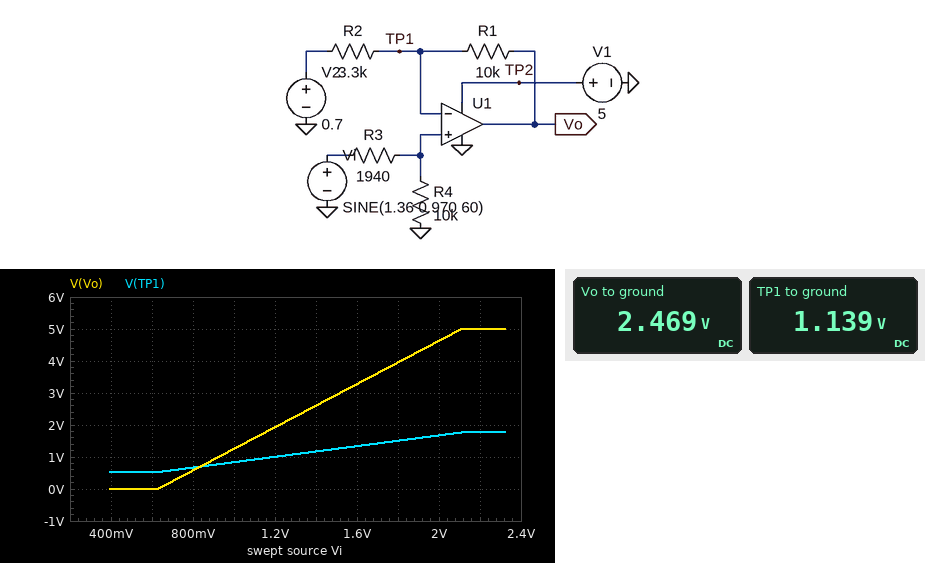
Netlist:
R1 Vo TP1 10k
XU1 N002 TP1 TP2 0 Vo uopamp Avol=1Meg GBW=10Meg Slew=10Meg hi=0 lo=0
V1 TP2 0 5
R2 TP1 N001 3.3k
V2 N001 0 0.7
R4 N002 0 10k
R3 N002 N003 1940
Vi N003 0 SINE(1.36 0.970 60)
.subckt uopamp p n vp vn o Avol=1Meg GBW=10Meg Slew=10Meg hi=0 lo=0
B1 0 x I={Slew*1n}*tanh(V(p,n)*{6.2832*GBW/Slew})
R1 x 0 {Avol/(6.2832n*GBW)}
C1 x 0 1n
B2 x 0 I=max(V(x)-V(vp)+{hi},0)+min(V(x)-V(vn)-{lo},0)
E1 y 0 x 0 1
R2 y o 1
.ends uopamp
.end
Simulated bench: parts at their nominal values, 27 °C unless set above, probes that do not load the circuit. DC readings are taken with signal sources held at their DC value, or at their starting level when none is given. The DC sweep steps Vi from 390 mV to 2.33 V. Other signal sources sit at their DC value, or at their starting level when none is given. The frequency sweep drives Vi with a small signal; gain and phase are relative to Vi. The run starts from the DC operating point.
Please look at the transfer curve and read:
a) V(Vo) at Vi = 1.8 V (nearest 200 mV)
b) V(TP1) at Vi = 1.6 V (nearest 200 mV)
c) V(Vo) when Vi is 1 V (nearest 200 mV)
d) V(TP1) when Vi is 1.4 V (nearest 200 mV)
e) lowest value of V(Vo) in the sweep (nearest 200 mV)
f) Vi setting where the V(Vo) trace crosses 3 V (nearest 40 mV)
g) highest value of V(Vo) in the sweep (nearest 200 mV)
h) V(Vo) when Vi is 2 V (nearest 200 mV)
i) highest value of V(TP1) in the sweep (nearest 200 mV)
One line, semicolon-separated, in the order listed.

4.0 V; 1.4 V; 1.2 V; 1.2 V; 0 V; 1.52 V; 5.0 V; 4.6 V; 1.8 V
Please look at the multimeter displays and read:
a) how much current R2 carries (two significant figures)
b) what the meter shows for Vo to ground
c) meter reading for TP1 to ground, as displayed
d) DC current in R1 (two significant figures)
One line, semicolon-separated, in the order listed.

130 µA; 2.469 V; 1.139 V; 130 µA
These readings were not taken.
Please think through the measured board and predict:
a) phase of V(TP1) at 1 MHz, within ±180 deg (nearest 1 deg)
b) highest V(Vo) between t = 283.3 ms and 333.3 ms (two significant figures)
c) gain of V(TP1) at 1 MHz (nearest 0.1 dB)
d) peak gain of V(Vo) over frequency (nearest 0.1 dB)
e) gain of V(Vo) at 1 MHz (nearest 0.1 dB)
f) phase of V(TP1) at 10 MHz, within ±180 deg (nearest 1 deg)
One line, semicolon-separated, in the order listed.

-22 deg; 5.0 V; -2.2 dB; 10.6 dB; 9.9 dB; -76 deg
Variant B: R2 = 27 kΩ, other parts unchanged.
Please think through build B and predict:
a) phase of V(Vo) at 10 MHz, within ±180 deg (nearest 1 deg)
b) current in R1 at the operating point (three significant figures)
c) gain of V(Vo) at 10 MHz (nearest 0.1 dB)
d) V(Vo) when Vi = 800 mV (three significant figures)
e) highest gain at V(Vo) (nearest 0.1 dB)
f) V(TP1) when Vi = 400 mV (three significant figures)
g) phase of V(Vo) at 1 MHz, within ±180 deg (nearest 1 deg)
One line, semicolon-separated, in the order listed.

-54 deg; 16.3 µA; -3.4 dB; 659 mV; 1.2 dB; 335 mV; -8 deg
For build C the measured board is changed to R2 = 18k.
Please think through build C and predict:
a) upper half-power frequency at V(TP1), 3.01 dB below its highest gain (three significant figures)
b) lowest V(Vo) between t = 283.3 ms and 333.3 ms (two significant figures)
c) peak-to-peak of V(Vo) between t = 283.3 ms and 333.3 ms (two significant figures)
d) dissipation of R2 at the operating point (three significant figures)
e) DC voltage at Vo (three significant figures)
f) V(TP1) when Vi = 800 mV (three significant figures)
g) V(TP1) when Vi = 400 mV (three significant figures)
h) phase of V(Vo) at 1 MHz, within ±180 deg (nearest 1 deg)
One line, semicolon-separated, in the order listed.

6.43 MHz; 120 mV; 2.5 V; 10.7 µW; 1.38 V; 670 mV; 335 mV; -9 deg
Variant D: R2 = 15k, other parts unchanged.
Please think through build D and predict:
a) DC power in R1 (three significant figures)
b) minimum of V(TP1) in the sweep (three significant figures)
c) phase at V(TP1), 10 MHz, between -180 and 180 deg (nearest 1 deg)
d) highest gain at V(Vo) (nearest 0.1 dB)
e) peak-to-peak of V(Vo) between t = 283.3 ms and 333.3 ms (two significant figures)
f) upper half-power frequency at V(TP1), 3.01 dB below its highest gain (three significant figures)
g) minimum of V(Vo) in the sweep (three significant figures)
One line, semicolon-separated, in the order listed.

8.57 µW; 327 mV; -59 deg; 2.9 dB; 2.7 V; 6.00 MHz; 77.7 mV
